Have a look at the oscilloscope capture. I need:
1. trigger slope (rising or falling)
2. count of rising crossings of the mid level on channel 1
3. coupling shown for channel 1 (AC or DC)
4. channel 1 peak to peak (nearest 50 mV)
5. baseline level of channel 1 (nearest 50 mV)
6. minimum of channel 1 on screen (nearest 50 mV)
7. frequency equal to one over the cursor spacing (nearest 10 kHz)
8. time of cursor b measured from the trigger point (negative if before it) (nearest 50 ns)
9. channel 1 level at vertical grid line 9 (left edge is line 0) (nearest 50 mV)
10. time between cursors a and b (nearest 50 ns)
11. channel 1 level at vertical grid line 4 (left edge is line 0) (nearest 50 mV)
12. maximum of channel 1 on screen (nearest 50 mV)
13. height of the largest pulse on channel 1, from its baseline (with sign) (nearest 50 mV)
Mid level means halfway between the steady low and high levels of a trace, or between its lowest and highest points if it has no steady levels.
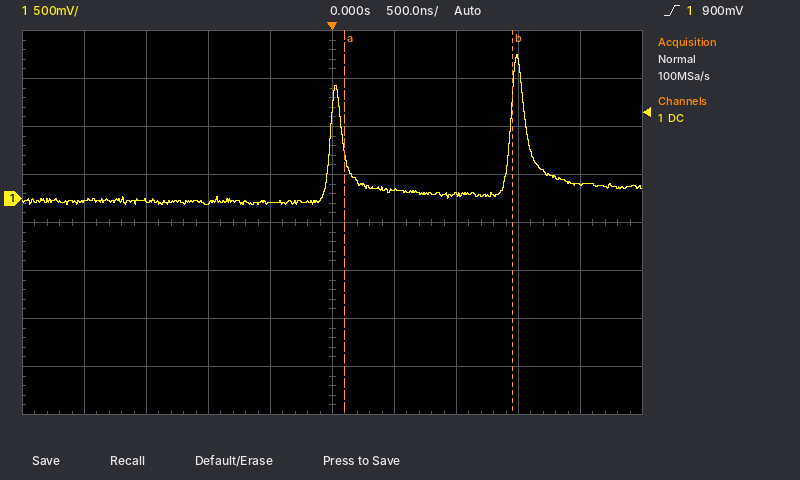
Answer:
rising
2
DC
1.55 V
0 mV
-50 mV
740 kHz
+1.45 µs
150 mV
1.35 µs
-50 mV
1.50 V
+1.50 V
